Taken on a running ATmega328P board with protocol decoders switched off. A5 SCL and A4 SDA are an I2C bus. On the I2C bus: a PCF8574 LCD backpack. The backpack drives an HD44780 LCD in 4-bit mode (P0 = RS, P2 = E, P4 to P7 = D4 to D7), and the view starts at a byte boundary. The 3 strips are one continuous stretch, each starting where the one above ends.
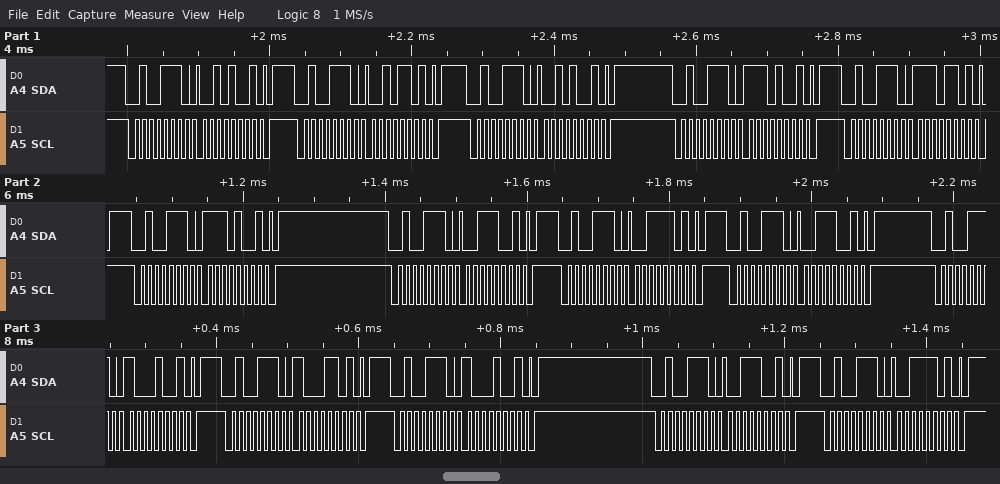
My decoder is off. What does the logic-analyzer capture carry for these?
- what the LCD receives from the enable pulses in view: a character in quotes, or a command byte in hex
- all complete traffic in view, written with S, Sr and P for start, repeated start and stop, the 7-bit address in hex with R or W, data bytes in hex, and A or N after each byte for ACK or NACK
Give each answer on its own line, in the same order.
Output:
'.' '8'
S 27W A 29 A P S 27W A 2D A P S 27W A 29 A P S 27W A E9 A P S 27W A ED A P S 27W A E9 A P S 27W A 39 A P S 27W A 3D A P S 27W A 39 A P S 27W A 89 A P S 27W A 8D A P S 27W A 89 A P S 27W A 39 A P S 27W A 3D A P
